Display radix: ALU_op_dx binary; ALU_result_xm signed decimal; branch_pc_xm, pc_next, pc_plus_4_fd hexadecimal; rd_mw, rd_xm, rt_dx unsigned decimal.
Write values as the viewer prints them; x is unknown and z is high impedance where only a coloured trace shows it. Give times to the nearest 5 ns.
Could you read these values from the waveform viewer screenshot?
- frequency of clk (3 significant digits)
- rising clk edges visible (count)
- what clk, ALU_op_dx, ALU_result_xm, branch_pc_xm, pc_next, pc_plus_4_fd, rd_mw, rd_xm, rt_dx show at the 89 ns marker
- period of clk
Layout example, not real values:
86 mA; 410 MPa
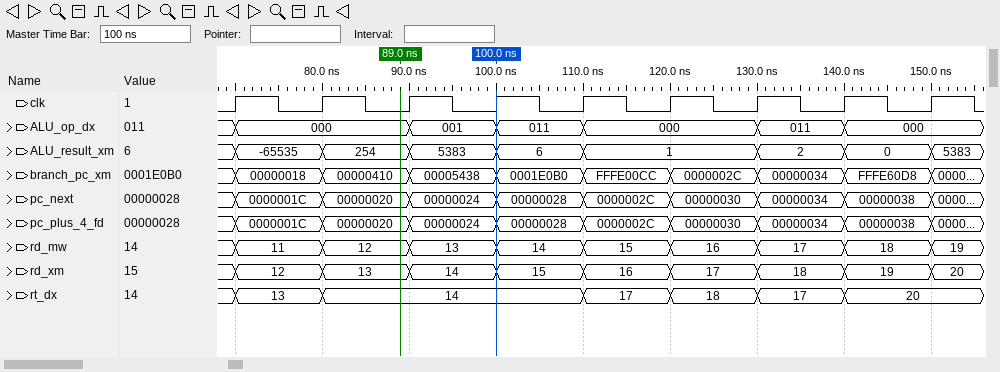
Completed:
100 MHz; 9; clk=0, ALU_op_dx=000, ALU_result_xm=254, branch_pc_xm=00000410, pc_next=00000020, pc_plus_4_fd=00000020, rd_mw=12, rd_xm=13, rt_dx=14; 10 ns
